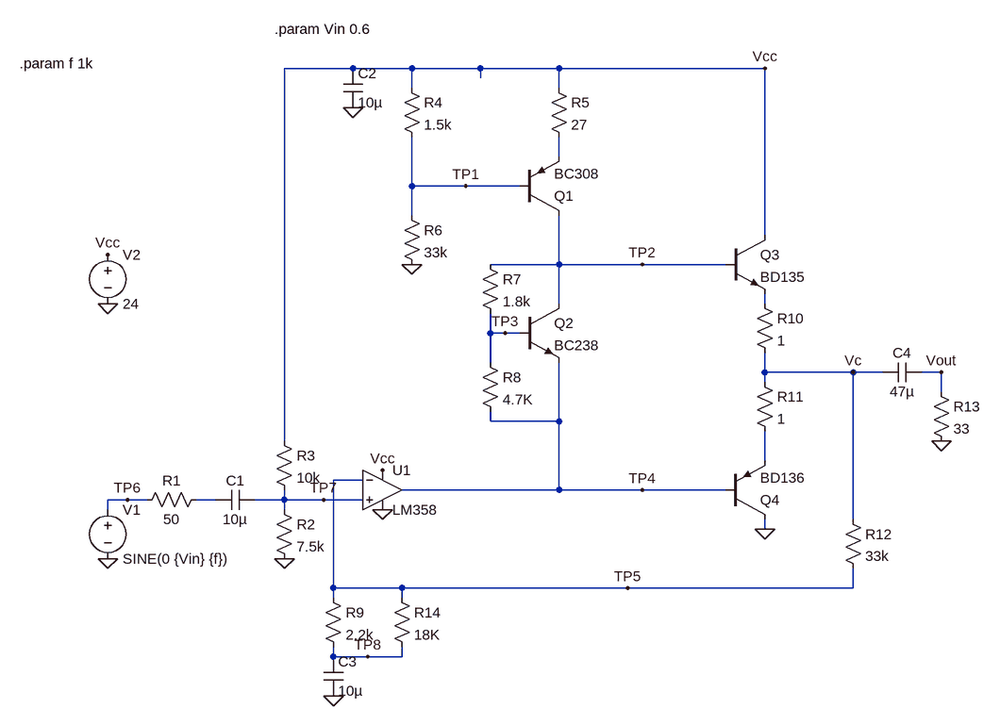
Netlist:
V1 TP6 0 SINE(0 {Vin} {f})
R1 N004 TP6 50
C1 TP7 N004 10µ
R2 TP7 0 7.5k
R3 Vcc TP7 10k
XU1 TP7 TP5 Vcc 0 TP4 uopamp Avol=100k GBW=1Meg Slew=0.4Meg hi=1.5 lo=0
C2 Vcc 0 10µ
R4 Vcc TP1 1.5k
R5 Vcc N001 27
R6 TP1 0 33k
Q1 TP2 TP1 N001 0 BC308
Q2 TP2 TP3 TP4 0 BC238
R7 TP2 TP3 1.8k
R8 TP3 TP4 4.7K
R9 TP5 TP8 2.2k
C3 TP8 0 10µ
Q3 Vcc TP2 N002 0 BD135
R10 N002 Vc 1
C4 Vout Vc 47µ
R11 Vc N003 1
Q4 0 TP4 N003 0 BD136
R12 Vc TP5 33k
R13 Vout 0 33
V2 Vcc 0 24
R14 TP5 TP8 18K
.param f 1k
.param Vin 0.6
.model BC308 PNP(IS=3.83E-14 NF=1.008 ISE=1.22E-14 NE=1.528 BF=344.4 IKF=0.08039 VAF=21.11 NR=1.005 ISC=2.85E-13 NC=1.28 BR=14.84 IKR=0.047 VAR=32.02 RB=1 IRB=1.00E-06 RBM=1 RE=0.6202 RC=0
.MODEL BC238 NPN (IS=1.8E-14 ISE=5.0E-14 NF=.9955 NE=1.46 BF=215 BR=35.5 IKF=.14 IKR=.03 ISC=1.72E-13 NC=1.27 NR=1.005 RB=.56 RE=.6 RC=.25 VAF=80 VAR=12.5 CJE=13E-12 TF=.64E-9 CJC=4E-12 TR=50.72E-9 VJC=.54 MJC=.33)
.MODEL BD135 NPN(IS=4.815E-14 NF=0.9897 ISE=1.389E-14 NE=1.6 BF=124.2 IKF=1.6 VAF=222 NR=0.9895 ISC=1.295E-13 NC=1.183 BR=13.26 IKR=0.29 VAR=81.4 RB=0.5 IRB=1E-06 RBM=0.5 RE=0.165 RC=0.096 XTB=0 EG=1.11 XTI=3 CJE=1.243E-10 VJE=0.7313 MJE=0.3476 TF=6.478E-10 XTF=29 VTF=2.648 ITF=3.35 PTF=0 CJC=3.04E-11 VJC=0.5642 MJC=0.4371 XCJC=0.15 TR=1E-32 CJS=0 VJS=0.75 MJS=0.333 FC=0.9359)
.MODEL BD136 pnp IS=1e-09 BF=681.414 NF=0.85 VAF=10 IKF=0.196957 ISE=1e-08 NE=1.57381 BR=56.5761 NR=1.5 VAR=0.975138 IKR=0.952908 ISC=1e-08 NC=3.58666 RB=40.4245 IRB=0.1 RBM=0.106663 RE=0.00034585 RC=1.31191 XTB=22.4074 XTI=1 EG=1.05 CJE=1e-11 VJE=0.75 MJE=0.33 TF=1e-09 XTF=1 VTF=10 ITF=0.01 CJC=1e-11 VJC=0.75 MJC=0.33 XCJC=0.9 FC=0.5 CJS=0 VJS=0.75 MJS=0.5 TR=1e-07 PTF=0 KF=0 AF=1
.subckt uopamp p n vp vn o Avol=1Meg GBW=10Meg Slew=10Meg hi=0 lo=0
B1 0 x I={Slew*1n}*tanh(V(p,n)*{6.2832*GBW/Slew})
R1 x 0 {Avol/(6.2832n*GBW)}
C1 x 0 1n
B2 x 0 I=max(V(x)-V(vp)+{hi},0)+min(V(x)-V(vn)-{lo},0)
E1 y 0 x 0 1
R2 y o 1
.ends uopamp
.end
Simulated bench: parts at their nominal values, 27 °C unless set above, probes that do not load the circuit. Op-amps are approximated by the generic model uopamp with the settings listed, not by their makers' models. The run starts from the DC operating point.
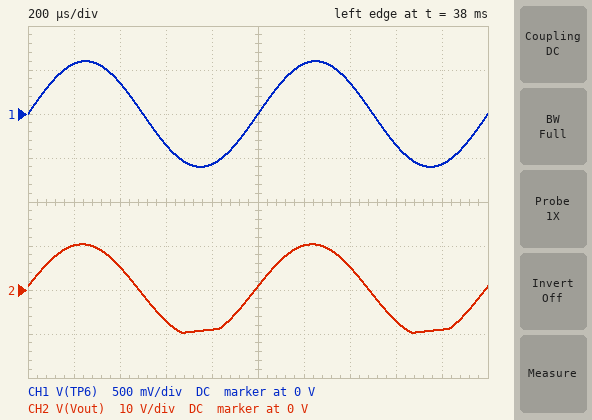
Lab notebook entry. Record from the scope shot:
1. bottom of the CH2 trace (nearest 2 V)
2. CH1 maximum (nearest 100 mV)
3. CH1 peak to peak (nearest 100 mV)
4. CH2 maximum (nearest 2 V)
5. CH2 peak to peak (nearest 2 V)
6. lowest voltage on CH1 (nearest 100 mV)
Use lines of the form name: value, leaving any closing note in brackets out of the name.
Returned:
bottom of the CH2 trace: -10 V
CH1 maximum: 600 mV
CH1 peak to peak: 1.2 V
CH2 maximum: 10 V
CH2 peak to peak: 20 V
lowest voltage on CH1: -600 mV
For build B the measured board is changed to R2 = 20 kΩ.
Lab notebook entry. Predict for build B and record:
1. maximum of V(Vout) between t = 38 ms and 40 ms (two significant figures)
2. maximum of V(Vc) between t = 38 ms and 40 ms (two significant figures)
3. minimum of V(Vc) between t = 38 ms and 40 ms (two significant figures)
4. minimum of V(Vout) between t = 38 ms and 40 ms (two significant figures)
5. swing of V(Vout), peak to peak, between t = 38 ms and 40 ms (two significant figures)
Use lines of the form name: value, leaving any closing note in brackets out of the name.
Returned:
maximum of V(Vout) between t = 38 ms and 40 ms: 7.4 V
maximum of V(Vc) between t = 38 ms and 40 ms: 23 V
minimum of V(Vc) between t = 38 ms and 40 ms: 6.1 V
minimum of V(Vout) between t = 38 ms and 40 ms: -9.6 V
swing of V(Vout), peak to peak, between t = 38 ms and 40 ms: 17 V
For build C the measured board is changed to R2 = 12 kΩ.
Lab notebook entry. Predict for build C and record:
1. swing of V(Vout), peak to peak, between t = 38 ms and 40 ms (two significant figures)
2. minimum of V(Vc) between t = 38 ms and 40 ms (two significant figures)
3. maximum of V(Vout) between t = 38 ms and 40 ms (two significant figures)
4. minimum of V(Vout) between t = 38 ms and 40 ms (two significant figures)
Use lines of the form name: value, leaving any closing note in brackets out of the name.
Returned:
swing of V(Vout), peak to peak, between t = 38 ms and 40 ms: 20 V
minimum of V(Vc) between t = 38 ms and 40 ms: 2.6 V
maximum of V(Vout) between t = 38 ms and 40 ms: 9.8 V
minimum of V(Vout) between t = 38 ms and 40 ms: -10 V
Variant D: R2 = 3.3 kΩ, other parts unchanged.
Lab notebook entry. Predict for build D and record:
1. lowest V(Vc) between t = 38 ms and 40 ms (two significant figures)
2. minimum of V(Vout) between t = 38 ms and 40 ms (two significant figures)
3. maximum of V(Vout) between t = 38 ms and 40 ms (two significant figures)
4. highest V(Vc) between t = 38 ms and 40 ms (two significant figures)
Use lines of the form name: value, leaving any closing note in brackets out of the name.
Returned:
lowest V(Vc) between t = 38 ms and 40 ms: 670 mV
minimum of V(Vout) between t = 38 ms and 40 ms: -6.2 V
maximum of V(Vout) between t = 38 ms and 40 ms: 8.9 V
highest V(Vc) between t = 38 ms and 40 ms: 15 V
